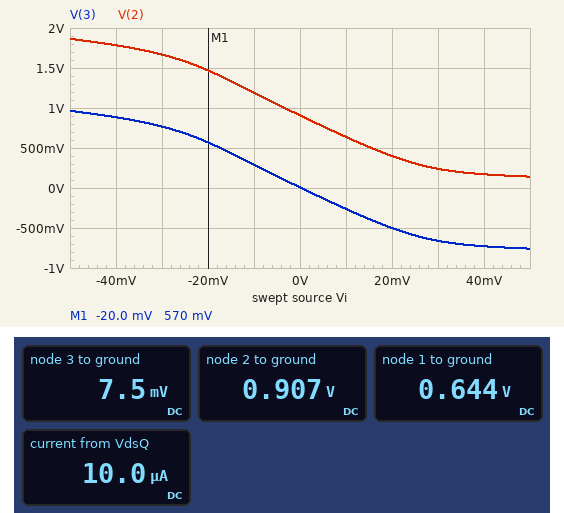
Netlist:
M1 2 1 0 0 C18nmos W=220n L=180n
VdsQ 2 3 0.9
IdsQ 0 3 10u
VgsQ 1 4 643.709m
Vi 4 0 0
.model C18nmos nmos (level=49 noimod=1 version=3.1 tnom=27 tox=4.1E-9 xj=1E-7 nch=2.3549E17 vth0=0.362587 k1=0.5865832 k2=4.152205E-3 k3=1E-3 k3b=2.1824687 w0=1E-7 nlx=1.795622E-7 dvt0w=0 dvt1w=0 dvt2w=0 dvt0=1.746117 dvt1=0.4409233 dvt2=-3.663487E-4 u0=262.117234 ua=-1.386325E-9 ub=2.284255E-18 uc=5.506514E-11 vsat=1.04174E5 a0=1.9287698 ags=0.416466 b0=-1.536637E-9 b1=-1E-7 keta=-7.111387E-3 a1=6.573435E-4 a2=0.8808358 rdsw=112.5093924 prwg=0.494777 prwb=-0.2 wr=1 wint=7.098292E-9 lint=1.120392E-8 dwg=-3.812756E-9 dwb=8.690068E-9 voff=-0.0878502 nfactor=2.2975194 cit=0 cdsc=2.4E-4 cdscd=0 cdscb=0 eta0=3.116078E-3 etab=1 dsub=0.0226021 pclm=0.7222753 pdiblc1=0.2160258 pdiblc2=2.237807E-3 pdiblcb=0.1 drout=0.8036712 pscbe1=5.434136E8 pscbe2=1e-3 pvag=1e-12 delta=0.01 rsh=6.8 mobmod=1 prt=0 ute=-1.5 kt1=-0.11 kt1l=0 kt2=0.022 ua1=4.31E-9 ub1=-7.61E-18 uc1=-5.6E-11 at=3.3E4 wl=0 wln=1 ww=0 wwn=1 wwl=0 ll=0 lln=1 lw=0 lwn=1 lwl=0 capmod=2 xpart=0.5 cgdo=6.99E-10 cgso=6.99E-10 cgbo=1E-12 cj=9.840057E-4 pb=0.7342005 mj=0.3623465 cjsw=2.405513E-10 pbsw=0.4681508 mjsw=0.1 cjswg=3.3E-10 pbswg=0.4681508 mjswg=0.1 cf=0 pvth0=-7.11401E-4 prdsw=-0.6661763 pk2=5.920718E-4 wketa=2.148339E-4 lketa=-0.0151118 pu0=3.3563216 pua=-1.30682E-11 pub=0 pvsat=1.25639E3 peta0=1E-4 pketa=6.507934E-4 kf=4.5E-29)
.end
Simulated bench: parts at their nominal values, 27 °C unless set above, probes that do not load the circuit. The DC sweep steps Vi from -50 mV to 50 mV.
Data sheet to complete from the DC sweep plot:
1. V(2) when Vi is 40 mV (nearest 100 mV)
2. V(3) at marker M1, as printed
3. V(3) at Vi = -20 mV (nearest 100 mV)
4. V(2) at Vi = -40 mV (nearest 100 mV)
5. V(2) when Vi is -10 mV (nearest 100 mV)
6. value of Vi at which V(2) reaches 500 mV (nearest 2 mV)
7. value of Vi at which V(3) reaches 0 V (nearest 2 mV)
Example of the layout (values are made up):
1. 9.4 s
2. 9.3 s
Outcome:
1. 200 mV
2. 570 mV
3. 600 mV
4. 1.8 V
5. 1.2 V
6. 16 mV
7. 0 V
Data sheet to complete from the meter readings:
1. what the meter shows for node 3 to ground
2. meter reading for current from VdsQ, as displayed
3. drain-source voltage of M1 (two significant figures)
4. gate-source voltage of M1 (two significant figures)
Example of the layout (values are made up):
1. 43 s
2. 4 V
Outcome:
1. 7.5 mV
2. 10.0 µA
3. 910 mV
4. 640 mV
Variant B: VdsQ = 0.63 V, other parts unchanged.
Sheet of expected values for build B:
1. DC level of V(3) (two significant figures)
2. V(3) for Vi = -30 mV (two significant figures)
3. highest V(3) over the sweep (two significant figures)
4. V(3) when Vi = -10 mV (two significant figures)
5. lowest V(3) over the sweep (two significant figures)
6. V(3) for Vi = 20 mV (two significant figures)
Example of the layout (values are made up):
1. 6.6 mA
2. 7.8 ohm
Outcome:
1. 280 mV
2. 1.0 V
3. 1.2 V
4. 560 mV
5. -490 mV
6. -230 mV
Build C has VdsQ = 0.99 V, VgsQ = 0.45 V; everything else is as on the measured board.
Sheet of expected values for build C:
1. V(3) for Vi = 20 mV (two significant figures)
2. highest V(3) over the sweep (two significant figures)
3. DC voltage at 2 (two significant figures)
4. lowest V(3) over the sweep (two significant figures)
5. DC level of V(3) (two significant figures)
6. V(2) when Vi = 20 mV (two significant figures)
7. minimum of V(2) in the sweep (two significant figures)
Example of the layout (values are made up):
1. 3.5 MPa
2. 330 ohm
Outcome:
1. 1.4 V
2. 1.8 V
3. 2.5 V
4. 1.3 V
5. 1.5 V
6. 2.4 V
7. 2.3 V
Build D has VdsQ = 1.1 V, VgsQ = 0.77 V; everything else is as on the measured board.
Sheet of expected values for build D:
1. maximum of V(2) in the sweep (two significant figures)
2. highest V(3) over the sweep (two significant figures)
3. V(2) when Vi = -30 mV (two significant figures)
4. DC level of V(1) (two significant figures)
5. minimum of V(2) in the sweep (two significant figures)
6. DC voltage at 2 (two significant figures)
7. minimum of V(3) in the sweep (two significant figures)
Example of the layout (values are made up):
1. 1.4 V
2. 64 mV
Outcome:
1. 110 mV
2. -990 mV
3. 92 mV
4. 770 mV
5. 62 mV
6. 77 mV
7. -1.0 V
